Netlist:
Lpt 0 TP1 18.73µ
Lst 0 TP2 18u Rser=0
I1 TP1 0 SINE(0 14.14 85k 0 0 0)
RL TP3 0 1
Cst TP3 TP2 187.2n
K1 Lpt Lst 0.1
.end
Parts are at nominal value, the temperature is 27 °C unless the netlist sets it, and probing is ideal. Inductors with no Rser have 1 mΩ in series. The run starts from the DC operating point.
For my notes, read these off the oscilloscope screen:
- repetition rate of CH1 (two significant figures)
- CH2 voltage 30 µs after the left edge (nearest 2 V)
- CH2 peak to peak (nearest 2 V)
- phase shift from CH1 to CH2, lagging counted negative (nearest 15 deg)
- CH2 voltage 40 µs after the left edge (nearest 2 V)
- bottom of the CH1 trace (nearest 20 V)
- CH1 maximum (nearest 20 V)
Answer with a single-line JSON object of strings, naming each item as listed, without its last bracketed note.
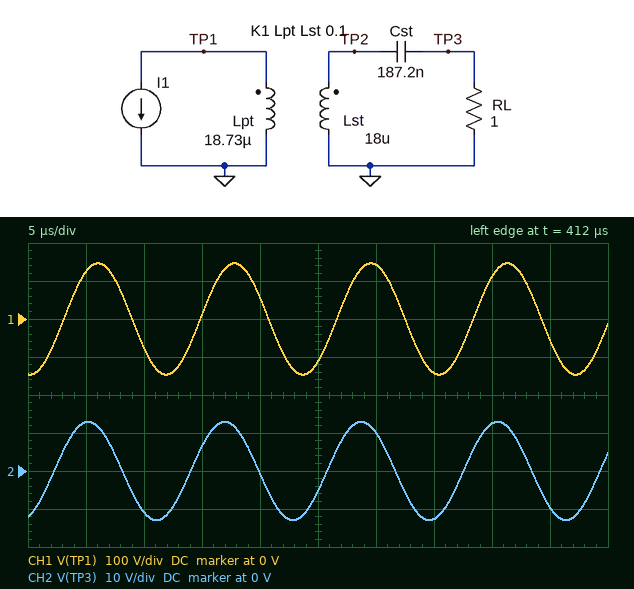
{"repetition rate of CH1": "85 kHz", "CH2 voltage 30 µs after the left edge": "10 V", "CH2 peak to peak": "26 V", "phase shift from CH1 to CH2, lagging counted negative": "30 deg", "CH2 voltage 40 µs after the left edge": "12 V", "bottom of the CH1 trace": "-140 V", "CH1 maximum": "140 V"}
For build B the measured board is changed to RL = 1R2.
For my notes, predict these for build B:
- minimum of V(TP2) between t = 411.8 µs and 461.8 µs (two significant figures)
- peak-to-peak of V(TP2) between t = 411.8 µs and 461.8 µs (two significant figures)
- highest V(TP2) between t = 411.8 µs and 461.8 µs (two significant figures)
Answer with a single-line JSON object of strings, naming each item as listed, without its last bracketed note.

{"minimum of V(TP2) between t = 411.8 µs and 461.8 µs": "-110 V", "peak-to-peak of V(TP2) between t = 411.8 µs and 461.8 µs": "220 V", "highest V(TP2) between t = 411.8 µs and 461.8 µs": "110 V"}
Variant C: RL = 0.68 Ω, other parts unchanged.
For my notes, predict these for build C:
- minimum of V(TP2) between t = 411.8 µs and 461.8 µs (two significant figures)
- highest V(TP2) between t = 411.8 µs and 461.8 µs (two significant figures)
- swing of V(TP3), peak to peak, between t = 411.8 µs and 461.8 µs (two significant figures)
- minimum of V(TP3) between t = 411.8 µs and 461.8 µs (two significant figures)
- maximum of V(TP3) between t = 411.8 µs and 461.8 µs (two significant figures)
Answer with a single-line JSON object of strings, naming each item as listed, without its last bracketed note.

{"minimum of V(TP2) between t = 411.8 µs and 461.8 µs": "-180 V", "highest V(TP2) between t = 411.8 µs and 461.8 µs": "180 V", "swing of V(TP3), peak to peak, between t = 411.8 µs and 461.8 µs": "24 V", "minimum of V(TP3) between t = 411.8 µs and 461.8 µs": "-12 V", "maximum of V(TP3) between t = 411.8 µs and 461.8 µs": "12 V"}
